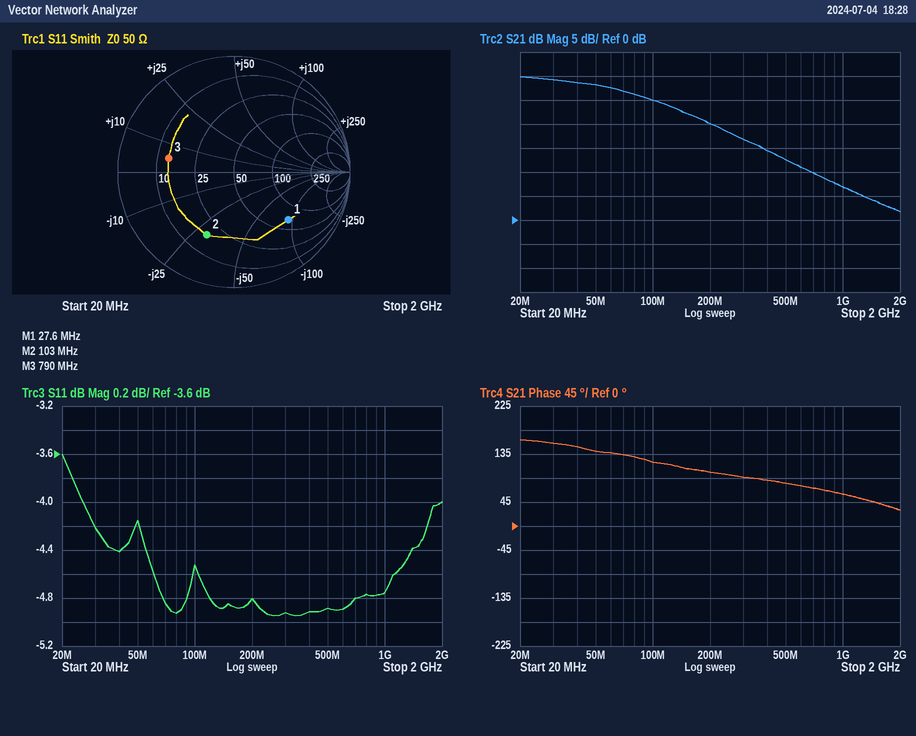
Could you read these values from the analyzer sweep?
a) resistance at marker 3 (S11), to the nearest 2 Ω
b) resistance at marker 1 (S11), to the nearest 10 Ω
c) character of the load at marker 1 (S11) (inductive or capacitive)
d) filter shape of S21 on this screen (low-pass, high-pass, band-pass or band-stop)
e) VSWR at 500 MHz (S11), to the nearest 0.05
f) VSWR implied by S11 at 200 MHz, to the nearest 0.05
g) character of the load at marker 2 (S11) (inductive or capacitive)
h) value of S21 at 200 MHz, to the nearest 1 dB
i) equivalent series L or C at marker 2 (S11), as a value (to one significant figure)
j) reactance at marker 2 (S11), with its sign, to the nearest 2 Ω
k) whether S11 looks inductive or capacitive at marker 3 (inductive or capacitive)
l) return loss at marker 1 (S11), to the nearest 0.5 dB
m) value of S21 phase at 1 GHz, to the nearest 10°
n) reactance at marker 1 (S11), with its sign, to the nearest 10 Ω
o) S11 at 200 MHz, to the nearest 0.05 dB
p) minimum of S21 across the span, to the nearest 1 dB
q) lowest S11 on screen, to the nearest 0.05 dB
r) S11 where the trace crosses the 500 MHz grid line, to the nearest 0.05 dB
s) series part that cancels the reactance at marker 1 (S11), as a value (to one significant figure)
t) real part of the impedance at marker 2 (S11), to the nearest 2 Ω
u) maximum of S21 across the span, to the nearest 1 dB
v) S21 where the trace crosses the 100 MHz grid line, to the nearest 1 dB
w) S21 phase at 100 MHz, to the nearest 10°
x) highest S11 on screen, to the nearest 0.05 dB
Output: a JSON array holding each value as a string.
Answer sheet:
["14 Ω", "70 Ω", "capacitive", "low-pass", "3.65", "3.70", "capacitive", "20 dB", "50 pF", "-30 Ω", "inductive", "4.0 dB", "60°", "-90 Ω", "-4.80 dB", "2 dB", "-4.95 dB", "-4.90 dB", "500 nH", "18 Ω", "30 dB", "25 dB", "120°", "-3.60 dB"]
